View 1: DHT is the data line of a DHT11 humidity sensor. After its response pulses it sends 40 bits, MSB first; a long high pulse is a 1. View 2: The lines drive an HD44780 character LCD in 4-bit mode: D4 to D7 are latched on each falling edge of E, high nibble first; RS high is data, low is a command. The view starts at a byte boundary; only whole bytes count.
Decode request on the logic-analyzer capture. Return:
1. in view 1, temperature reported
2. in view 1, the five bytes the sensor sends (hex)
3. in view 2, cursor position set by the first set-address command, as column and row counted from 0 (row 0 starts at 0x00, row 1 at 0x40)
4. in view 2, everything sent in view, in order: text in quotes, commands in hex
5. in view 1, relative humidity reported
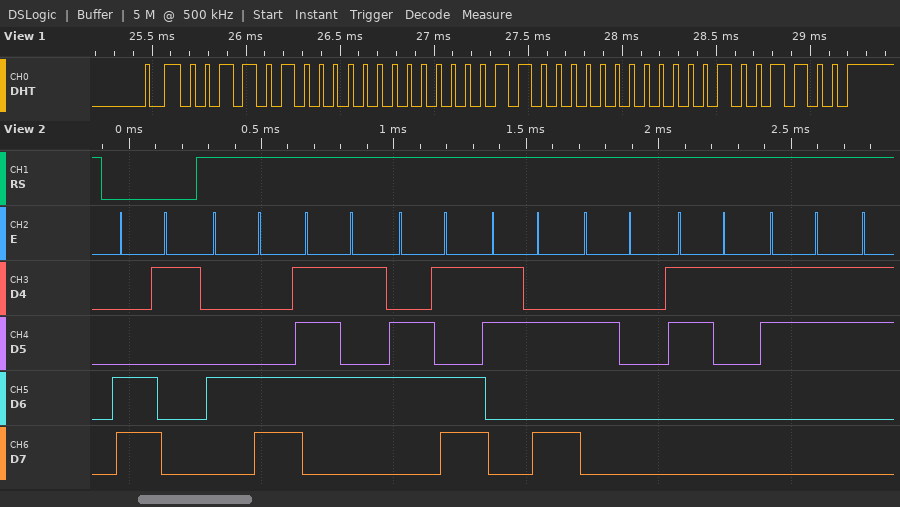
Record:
24.0 °C
34 00 18 00 4C
column 1, row 1
0xC1 "Lum: 13"
52 %
